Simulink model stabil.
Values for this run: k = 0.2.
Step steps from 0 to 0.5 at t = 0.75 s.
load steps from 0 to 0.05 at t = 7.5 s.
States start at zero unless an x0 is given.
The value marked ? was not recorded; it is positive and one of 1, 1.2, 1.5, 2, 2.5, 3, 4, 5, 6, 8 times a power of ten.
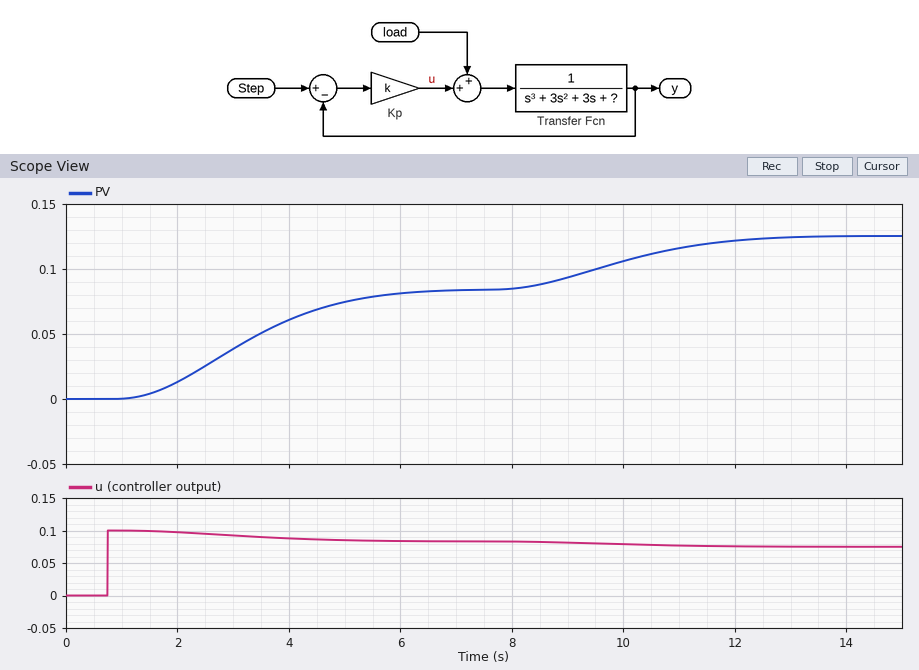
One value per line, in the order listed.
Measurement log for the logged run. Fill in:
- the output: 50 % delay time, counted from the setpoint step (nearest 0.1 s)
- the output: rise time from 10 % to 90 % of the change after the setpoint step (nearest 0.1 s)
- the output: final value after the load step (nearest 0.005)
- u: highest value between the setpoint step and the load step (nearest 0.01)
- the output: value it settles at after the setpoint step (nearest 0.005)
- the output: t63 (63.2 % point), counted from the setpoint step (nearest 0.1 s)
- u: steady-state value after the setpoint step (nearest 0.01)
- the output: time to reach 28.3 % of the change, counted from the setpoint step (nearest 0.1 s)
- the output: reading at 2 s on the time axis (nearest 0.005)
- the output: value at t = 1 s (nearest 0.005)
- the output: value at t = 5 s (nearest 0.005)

2.4 s
3.3 s
0.125
0.10
0.085
2.8 s
0.08
1.7 s
0.015
0.000
0.075
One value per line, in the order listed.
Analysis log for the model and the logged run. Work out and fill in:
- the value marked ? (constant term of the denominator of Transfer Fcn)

1
